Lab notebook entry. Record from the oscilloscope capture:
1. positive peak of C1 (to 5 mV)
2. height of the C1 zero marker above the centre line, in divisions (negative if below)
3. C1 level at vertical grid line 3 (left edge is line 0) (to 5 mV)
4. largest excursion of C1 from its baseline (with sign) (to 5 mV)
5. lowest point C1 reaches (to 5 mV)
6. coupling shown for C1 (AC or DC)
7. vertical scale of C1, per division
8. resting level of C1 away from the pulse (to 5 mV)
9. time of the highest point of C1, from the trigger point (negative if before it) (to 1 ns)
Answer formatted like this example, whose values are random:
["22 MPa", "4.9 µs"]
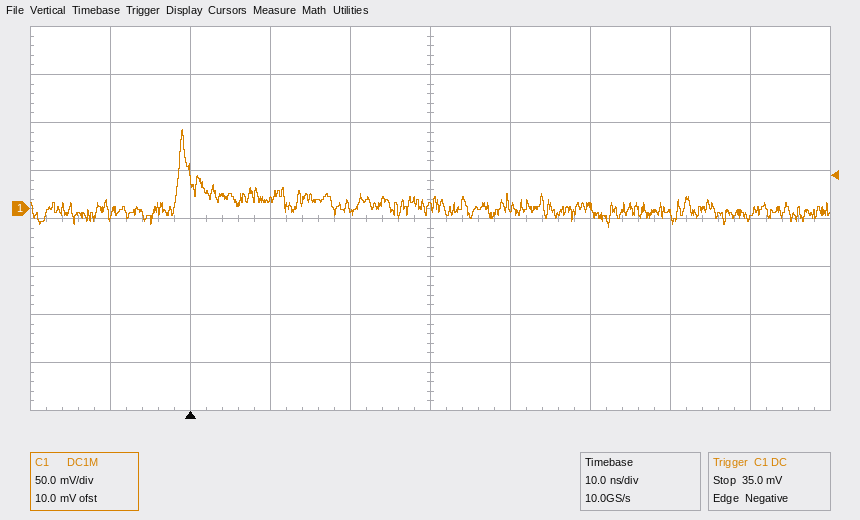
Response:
["85 mV", "+0.2 div", "10 mV", "+85 mV", "-20 mV", "DC", "50 mV", "0 mV", "-1 ns"]
